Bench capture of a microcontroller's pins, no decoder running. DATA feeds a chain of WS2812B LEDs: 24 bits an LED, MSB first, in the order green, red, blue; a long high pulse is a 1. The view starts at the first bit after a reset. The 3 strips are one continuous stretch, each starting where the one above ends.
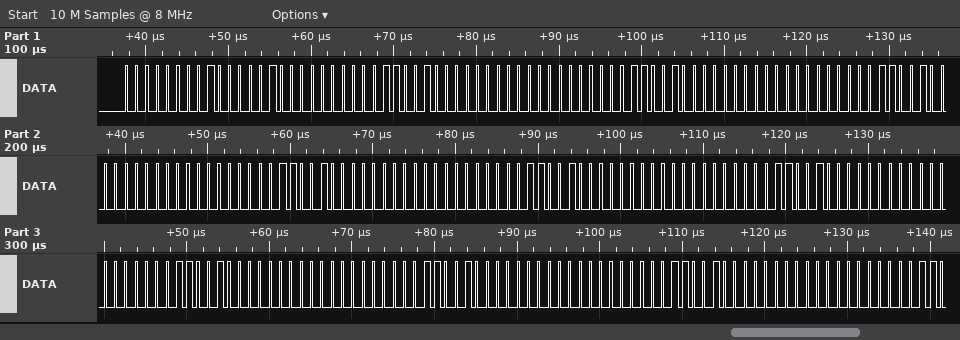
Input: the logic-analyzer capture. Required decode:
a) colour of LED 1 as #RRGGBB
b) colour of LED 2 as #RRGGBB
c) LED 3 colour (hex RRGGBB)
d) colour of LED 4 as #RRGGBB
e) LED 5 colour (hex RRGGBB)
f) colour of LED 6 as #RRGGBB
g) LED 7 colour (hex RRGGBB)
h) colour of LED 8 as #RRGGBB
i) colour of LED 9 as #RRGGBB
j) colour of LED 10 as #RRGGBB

#820000
#006400
#006400
#006400
#006400
#006400
#006400
#006400
#006400
#006400
